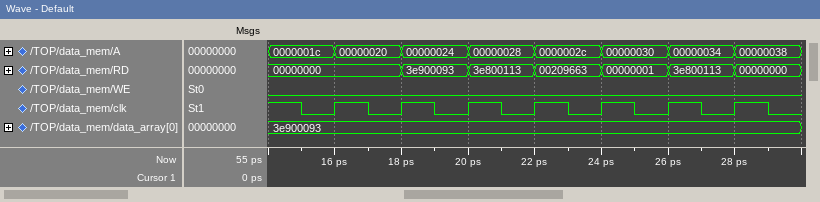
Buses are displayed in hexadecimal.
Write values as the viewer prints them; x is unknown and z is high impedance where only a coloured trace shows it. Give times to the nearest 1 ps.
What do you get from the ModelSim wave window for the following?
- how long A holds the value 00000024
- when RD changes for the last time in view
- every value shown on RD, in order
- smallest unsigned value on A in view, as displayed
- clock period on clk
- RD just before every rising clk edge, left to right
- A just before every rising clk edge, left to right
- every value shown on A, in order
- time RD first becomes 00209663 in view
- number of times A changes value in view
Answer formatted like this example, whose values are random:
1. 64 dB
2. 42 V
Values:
1. 2 ps
2. 28 ps
3. 00000000, 3e900093, 3e800113, 00209663, 00000001, 3e800113, 00000000
4. 0000001c
5. 2 ps
6. 00000000, 00000000, 3e900093, 3e800113, 00209663, 00000001, 3e800113
7. 0000001c, 00000020, 00000024, 00000028, 0000002c, 00000030, 00000034
8. 0000001c, 00000020, 00000024, 00000028, 0000002c, 00000030, 00000034, 00000038
9. 22 ps
10. 7
